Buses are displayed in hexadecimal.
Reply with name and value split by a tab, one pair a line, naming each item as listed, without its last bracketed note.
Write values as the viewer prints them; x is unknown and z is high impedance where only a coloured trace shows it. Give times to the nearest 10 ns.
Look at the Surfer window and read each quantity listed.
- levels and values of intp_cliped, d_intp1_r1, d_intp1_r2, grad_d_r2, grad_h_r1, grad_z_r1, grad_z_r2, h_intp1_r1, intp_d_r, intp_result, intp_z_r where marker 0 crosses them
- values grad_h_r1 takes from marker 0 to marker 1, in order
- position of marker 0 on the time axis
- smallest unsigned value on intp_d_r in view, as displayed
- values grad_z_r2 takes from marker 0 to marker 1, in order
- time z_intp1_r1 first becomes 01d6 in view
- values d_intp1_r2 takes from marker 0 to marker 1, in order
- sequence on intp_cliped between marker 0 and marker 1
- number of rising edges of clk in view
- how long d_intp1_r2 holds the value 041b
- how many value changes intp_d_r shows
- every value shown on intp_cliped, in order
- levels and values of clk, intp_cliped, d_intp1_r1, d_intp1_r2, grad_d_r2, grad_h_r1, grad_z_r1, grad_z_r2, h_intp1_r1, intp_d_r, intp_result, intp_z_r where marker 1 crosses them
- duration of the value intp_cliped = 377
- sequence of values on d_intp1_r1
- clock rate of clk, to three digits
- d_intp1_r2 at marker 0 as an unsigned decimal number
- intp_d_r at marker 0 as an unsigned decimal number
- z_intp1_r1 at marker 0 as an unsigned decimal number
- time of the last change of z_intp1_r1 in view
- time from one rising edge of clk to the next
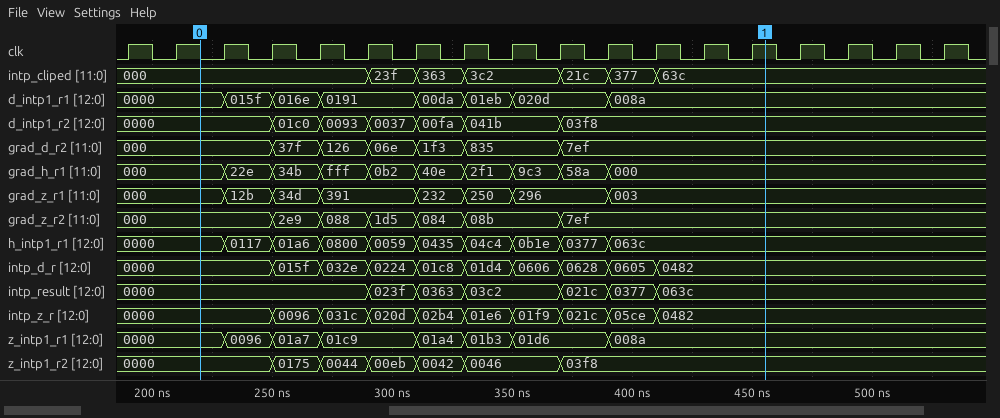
levels and values of intp_cliped, d_intp1_r1, d_intp1_r2, grad_d_r2, grad_h_r1, grad_z_r1, grad_z_r2, h_intp1_r1, intp_d_r, intp_result, intp_z_r where marker 0 crosses them	intp_cliped=000, d_intp1_r1=0000, d_intp1_r2=0000, grad_d_r2=000, grad_h_r1=000, grad_z_r1=000, grad_z_r2=000, h_intp1_r1=0000, intp_d_r=0000, intp_result=0000, intp_z_r=0000
values grad_h_r1 takes from marker 0 to marker 1, in order	000, 22e, 34b, fff, 0b2, 40e, 2f1, 9c3, 58a, 000
position of marker 0 on the time axis	220 ns
smallest unsigned value on intp_d_r in view, as displayed	0000
values grad_z_r2 takes from marker 0 to marker 1, in order	000, 2e9, 088, 1d5, 084, 08b, 7ef
time z_intp1_r1 first becomes 01d6 in view	350 ns
values d_intp1_r2 takes from marker 0 to marker 1, in order	0000, 01c0, 0093, 0037, 00fa, 041b, 03f8
sequence on intp_cliped between marker 0 and marker 1	000, 23f, 363, 3c2, 21c, 377, 63c
number of rising edges of clk in view	18
how long d_intp1_r2 holds the value 041b	40 ns
how many value changes intp_d_r shows	9
every value shown on intp_cliped, in order	000, 23f, 363, 3c2, 21c, 377, 63c
levels and values of clk, intp_cliped, d_intp1_r1, d_intp1_r2, grad_d_r2, grad_h_r1, grad_z_r1, grad_z_r2, h_intp1_r1, intp_d_r, intp_result, intp_z_r where marker 1 crosses them	clk=1, intp_cliped=63c, d_intp1_r1=008a, d_intp1_r2=03f8, grad_d_r2=7ef, grad_h_r1=000, grad_z_r1=003, grad_z_r2=7ef, h_intp1_r1=063c, intp_d_r=0482, intp_result=063c, intp_z_r=0482
duration of the value intp_cliped = 377	20 ns
sequence of values on d_intp1_r1	0000, 015f, 016e, 0191, 00da, 01eb, 020d, 008a
clock rate of clk, to three digits	50.0 MHz
d_intp1_r2 at marker 0 as an unsigned decimal number	0
intp_d_r at marker 0 as an unsigned decimal number	0
z_intp1_r1 at marker 0 as an unsigned decimal number	0
time of the last change of z_intp1_r1 in view	390 ns
time from one rising edge of clk to the next	20 ns
